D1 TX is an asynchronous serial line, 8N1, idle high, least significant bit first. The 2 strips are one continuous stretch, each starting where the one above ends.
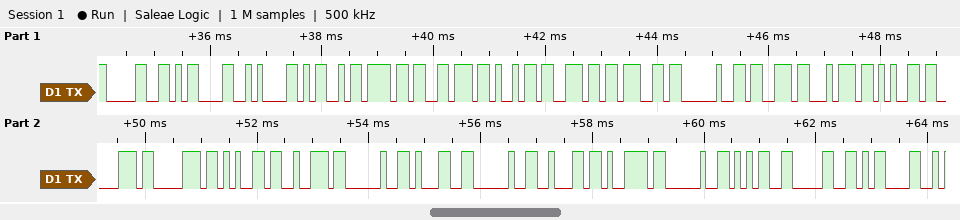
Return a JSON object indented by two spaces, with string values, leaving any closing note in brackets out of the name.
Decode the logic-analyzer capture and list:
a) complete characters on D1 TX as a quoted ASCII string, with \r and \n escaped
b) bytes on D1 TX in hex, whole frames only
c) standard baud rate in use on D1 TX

{
  "complete characters on D1 TX as a quoted ASCII string, with \\r and \\n escaped": "\"0\\r\\nMoving stepper 1 by 50\\r\"",
  "bytes on D1 TX in hex, whole frames only": "30 0D 0A 4D 6F 76 69 6E 67 20 73 74 65 70 70 65 72 20 31 20 62 79 20 35 30 0D",
  "standard baud rate in use on D1 TX": "9600 baud"
}
